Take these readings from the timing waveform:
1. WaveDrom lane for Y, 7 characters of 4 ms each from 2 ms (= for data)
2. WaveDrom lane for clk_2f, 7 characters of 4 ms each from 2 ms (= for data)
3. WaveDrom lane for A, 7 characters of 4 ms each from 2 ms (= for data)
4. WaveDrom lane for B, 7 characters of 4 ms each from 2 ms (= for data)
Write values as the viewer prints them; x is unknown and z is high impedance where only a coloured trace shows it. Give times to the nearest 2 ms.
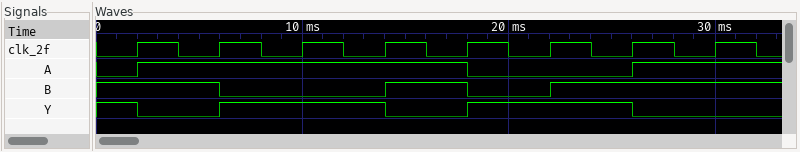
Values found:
{name: 'Y', wave: '01.01.0'}
{name: 'clk_2f', wave: 'p......'}
{name: 'A', wave: '1...0.1'}
{name: 'B', wave: '10.101.'}
